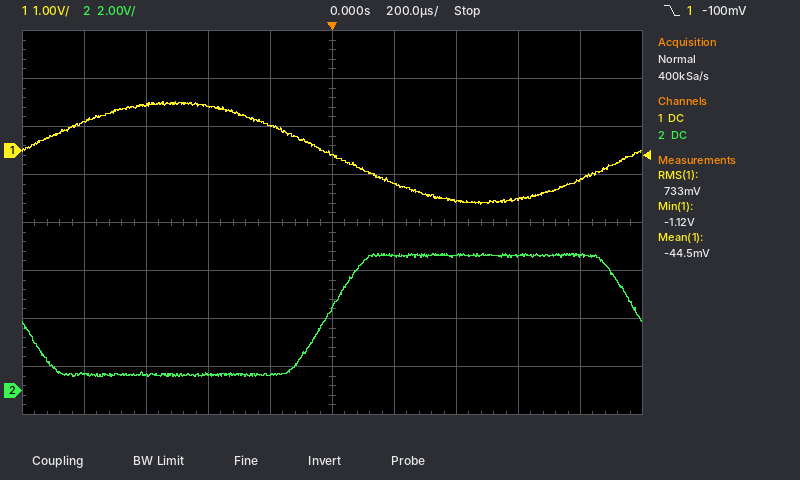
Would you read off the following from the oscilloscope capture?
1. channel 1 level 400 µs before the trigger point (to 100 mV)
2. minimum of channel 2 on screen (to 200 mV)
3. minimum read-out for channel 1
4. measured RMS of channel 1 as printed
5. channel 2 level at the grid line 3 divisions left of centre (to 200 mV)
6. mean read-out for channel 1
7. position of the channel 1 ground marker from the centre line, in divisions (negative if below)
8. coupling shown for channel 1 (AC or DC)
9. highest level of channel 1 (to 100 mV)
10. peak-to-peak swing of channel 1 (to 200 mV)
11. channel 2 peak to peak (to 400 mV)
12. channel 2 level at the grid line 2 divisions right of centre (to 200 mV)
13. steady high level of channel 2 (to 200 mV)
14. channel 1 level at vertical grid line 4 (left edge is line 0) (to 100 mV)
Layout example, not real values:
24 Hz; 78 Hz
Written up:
900 mV; 600 mV; -1.12 V; 733 mV; 600 mV; -44.5 mV; +1.5 div; DC; 1.0 V; 2.2 V; 5.2 V; 5.6 V; 5.6 V; 500 mV
